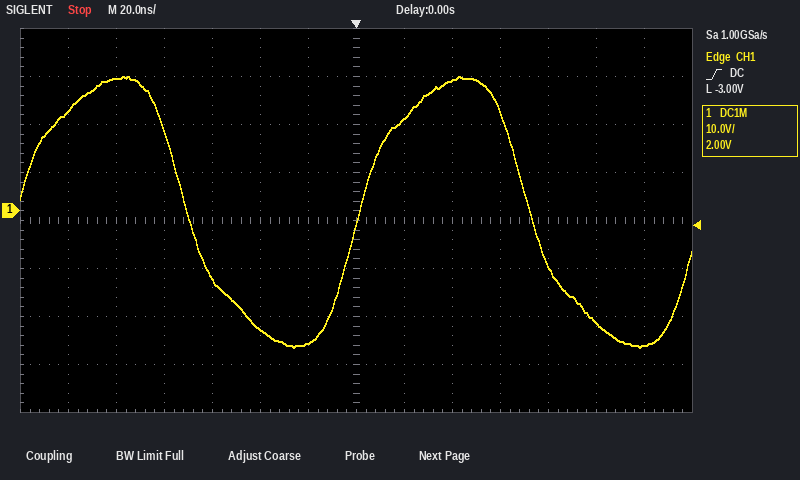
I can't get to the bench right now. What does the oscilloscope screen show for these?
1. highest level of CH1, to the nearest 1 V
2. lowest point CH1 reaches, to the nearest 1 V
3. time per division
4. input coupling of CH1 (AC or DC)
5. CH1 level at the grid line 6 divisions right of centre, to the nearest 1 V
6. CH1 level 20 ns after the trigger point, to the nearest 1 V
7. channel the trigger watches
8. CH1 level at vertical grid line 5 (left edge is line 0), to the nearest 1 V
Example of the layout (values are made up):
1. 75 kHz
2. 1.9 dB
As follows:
1. 28 V
2. -28 V
3. 20 ns
4. DC
5. -28 V
6. 19 V
7. CH1
8. -25 V
